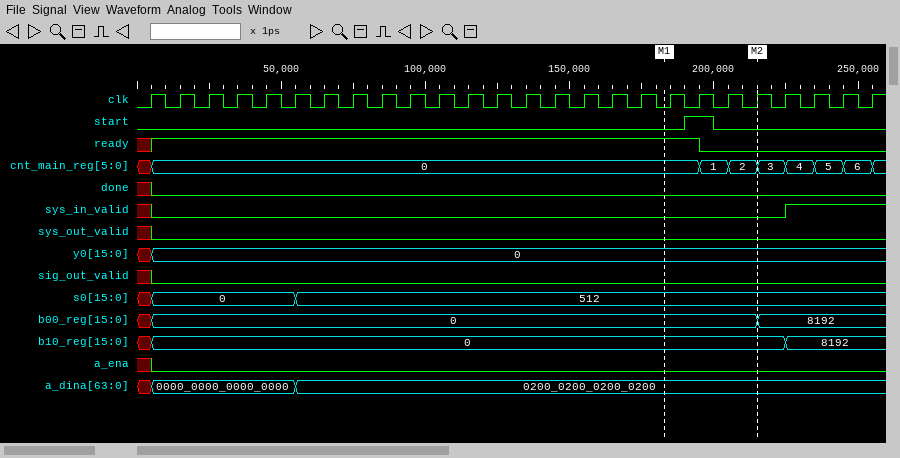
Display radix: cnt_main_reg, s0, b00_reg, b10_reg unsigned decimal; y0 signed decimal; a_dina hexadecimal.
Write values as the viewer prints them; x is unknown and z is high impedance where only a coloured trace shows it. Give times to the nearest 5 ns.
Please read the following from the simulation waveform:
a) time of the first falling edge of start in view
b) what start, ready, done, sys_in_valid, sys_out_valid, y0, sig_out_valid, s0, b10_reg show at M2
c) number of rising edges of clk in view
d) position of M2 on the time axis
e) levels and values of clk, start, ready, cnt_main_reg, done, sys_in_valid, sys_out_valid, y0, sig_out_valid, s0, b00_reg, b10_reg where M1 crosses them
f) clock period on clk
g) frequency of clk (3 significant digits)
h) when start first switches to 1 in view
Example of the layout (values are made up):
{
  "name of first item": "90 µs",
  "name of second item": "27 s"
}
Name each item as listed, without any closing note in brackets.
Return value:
{
  "time of the first falling edge of start in view": "200 ns",
  "what start, ready, done, sys_in_valid, sys_out_valid, y0, sig_out_valid, s0, b10_reg show at M2": "start=0, ready=0, done=0, sys_in_valid=0, sys_out_valid=0, y0=0, sig_out_valid=0, s0=512, b10_reg=0",
  "number of rising edges of clk in view": "26",
  "position of M2 on the time axis": "215 ns",
  "levels and values of clk, start, ready, cnt_main_reg, done, sys_in_valid, sys_out_valid, y0, sig_out_valid, s0, b00_reg, b10_reg where M1 crosses them": "clk=0, start=0, ready=1, cnt_main_reg=0, done=0, sys_in_valid=0, sys_out_valid=0, y0=0, sig_out_valid=0, s0=512, b00_reg=0, b10_reg=0",
  "clock period on clk": "10 ns",
  "frequency of clk": "100 MHz",
  "when start first switches to 1 in view": "190 ns"
}
